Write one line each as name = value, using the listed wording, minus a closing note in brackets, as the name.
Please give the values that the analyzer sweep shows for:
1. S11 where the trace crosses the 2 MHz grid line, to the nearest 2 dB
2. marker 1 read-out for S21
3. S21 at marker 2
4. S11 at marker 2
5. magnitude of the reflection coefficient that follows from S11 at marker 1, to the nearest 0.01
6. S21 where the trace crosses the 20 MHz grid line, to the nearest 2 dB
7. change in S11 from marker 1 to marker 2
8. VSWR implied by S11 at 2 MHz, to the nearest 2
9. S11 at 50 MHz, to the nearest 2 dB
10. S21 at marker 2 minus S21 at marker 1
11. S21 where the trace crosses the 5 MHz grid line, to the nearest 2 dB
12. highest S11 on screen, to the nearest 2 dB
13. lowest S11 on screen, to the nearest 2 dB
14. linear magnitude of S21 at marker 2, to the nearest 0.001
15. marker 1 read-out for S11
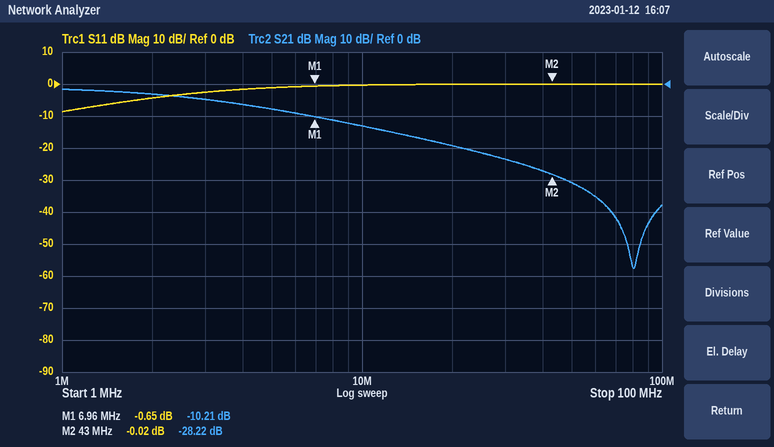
S11 where the trace crosses the 2 MHz grid line, to the nearest 2 dB = -4 dB
marker 1 read-out for S21 = -10.21 dB
S21 at marker 2 = -28.22 dB
S11 at marker 2 = -0.02 dB
magnitude of the reflection coefficient that follows from S11 at marker 1, to the nearest 0.01 = 0.93
S21 where the trace crosses the 20 MHz grid line, to the nearest 2 dB = -20 dB
change in S11 from marker 1 to marker 2 = 0.63 dB
VSWR implied by S11 at 2 MHz, to the nearest 2 = 4
S11 at 50 MHz, to the nearest 2 dB = 0 dB
S21 at marker 2 minus S21 at marker 1 = -18.01 dB
S21 where the trace crosses the 5 MHz grid line, to the nearest 2 dB = -8 dB
highest S11 on screen, to the nearest 2 dB = 0 dB
lowest S11 on screen, to the nearest 2 dB = -8 dB
linear magnitude of S21 at marker 2, to the nearest 0.001 = 0.039
marker 1 read-out for S11 = -0.65 dB
